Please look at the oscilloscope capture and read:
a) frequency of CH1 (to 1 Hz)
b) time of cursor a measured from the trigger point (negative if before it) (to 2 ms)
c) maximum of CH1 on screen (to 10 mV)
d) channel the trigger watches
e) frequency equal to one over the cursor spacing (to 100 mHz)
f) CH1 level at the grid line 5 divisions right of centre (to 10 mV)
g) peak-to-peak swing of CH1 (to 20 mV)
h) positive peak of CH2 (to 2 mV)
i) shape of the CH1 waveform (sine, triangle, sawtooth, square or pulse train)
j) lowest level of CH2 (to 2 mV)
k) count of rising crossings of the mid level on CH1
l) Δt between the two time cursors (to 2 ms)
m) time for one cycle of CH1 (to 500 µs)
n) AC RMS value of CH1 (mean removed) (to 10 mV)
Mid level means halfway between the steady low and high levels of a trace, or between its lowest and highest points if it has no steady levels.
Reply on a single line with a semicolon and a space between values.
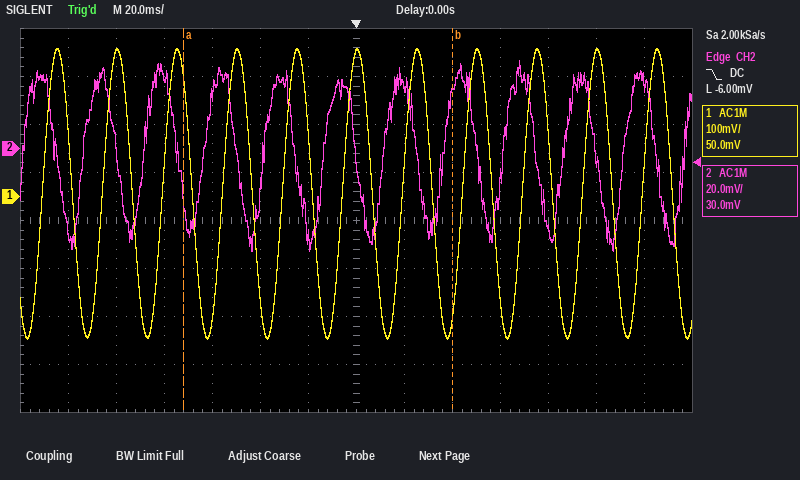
40 Hz; -72 ms; 310 mV; CH2; 8.9 Hz; 300 mV; 600 mV; 36 mV; sine; -42 mV; 11; 112 ms; 25.0 ms; 210 mV
